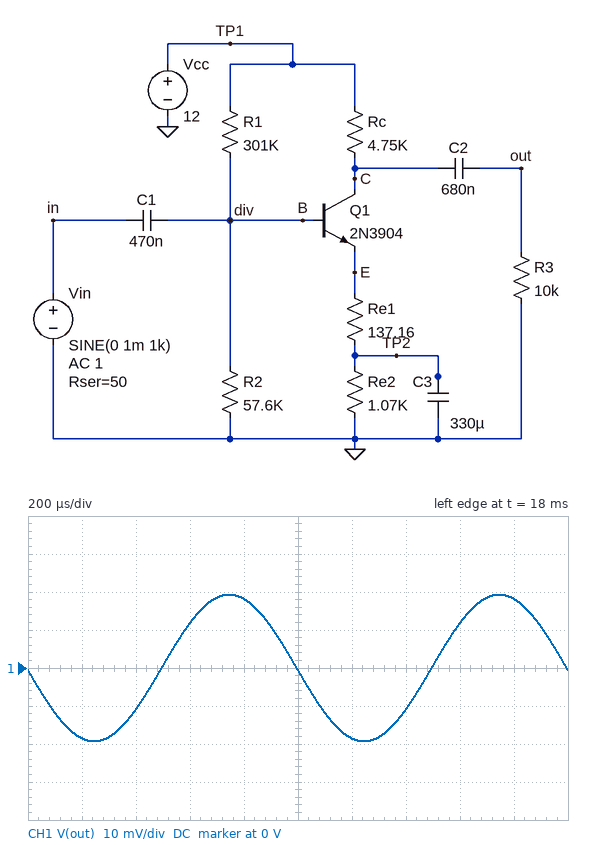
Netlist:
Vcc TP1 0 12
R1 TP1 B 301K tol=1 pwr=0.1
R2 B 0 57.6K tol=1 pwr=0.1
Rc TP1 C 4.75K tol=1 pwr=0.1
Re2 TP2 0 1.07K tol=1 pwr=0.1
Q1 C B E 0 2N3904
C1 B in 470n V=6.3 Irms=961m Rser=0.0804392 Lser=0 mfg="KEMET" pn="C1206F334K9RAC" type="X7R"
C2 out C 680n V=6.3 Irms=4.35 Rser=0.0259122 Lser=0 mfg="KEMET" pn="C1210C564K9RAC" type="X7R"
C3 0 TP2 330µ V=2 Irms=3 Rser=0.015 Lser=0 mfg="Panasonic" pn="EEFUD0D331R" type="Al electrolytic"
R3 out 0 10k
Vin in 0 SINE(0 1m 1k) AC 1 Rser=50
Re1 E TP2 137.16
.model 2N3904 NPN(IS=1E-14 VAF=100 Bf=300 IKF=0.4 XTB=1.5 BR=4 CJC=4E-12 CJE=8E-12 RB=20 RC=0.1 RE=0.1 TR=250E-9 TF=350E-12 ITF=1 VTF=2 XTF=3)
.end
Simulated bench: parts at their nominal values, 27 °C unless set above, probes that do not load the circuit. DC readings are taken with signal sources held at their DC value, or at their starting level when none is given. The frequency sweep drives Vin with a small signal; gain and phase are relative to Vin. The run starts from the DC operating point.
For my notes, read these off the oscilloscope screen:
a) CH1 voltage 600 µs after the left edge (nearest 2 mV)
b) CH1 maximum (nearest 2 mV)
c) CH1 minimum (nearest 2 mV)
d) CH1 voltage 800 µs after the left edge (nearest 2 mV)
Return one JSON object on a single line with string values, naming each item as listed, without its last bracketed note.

{"CH1 voltage 600 µs after the left edge": "12 mV", "CH1 maximum": "20 mV", "CH1 minimum": "-20 mV", "CH1 voltage 800 µs after the left edge": "18 mV"}
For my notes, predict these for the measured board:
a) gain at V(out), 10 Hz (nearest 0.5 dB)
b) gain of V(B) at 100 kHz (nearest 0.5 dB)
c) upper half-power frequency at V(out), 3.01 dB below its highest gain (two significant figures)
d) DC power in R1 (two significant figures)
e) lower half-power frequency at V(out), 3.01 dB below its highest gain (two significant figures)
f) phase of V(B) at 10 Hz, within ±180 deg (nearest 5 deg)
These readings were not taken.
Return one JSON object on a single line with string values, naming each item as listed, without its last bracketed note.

{"gain at V(out), 10 Hz": "15.0 dB", "gain of V(B) at 100 kHz": "0 dB", "upper half-power frequency at V(out), 3.01 dB below its highest gain": "17 MHz", "DC power in R1": "350 µW", "lower half-power frequency at V(out), 3.01 dB below its highest gain": "24 Hz", "phase of V(B) at 10 Hz, within ±180 deg": "50 deg"}
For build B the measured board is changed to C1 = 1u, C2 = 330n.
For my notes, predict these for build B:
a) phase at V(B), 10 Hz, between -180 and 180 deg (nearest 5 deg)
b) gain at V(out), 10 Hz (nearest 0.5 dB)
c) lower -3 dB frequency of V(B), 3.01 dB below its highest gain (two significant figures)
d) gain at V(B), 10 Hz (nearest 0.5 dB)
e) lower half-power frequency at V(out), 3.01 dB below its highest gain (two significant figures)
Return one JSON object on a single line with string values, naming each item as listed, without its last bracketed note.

{"phase at V(B), 10 Hz, between -180 and 180 deg": "30 deg", "gain at V(out), 10 Hz": "12.5 dB", "lower -3 dB frequency of V(B), 3.01 dB below its highest gain": "7.2 Hz", "gain at V(B), 10 Hz": "-2.0 dB", "lower half-power frequency at V(out), 3.01 dB below its highest gain": "35 Hz"}
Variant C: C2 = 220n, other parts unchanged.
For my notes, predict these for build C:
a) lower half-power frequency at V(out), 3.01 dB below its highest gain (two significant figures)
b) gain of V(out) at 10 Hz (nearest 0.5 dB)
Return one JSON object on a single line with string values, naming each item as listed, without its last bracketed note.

{"lower half-power frequency at V(out), 3.01 dB below its highest gain": "53 Hz", "gain of V(out) at 10 Hz": "6.5 dB"}
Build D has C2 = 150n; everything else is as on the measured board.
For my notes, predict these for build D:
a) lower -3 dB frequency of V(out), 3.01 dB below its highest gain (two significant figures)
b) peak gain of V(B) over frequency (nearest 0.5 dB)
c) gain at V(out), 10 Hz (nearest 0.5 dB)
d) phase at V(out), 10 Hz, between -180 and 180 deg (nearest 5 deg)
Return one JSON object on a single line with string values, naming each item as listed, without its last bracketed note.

{"lower -3 dB frequency of V(out), 3.01 dB below its highest gain": "75 Hz", "peak gain of V(B) over frequency": "0 dB", "gain at V(out), 10 Hz": "3.0 dB", "phase at V(out), 10 Hz, between -180 and 180 deg": "-35 deg"}
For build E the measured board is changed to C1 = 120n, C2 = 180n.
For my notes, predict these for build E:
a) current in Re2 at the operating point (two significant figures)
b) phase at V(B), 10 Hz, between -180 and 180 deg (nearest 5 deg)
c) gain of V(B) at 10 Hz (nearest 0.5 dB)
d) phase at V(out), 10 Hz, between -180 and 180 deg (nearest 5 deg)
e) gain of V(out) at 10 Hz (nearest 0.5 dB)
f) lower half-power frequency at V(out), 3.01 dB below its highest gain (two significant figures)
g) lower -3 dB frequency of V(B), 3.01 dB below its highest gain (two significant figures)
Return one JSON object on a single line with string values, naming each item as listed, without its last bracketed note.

{"current in Re2 at the operating point": "940 µA", "phase at V(B), 10 Hz, between -180 and 180 deg": "70 deg", "gain of V(B) at 10 Hz": "-14.5 dB", "phase at V(out), 10 Hz, between -180 and 180 deg": "-10 deg", "gain of V(out) at 10 Hz": "-5.0 dB", "lower half-power frequency at V(out), 3.01 dB below its highest gain": "89 Hz", "lower -3 dB frequency of V(B), 3.01 dB below its highest gain": "55 Hz"}
